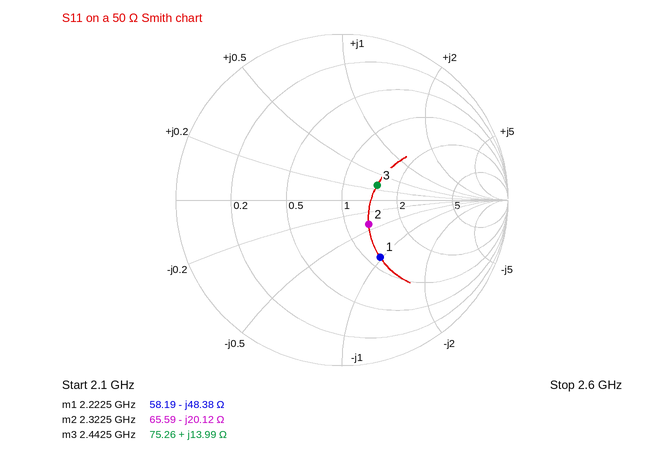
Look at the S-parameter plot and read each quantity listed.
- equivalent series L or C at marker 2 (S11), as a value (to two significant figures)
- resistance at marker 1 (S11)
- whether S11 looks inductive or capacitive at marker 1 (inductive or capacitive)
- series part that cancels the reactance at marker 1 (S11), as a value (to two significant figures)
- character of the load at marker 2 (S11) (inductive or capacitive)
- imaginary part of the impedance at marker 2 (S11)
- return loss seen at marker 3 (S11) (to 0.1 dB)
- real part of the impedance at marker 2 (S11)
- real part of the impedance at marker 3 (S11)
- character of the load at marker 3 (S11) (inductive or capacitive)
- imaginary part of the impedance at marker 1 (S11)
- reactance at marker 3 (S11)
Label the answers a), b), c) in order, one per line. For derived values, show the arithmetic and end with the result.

a) C = 1/(2π × 2.3225 GHz × 20.12 Ω) ≈ 3.4 pF
b) 58.19 Ω
c) capacitive
d) L = 48.38 Ω/(2π × 2.2225 GHz) ≈ 3.5 nH
e) capacitive
f) -20.12 Ω
g) 12.8 dB
h) 65.59 Ω
i) 75.26 Ω
j) inductive
k) -48.38 Ω
l) +13.99 Ω
